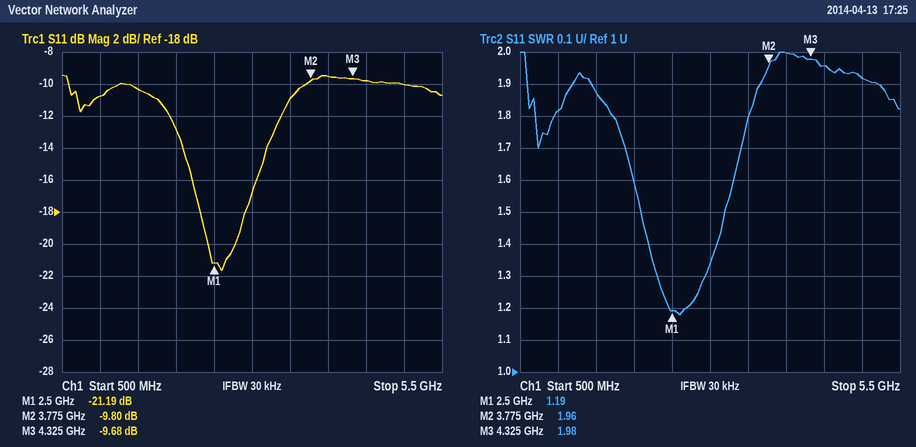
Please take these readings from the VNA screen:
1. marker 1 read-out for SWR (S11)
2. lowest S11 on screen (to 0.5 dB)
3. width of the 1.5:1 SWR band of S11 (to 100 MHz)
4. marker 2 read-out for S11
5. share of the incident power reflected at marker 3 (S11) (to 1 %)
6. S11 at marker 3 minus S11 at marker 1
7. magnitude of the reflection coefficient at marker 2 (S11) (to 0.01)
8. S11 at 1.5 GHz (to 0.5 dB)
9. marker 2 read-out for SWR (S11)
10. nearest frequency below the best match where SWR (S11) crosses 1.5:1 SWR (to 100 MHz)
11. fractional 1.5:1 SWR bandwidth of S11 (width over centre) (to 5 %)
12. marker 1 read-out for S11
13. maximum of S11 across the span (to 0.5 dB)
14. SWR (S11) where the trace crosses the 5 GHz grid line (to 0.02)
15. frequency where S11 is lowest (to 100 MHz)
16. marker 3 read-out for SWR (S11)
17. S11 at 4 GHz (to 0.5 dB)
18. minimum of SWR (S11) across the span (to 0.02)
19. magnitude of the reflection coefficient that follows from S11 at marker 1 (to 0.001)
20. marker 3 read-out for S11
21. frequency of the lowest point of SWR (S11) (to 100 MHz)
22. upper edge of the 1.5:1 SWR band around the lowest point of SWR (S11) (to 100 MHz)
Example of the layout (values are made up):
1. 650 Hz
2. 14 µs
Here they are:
1. 1.19
2. -21.5 dB
3. 1.1 GHz
4. -9.80 dB
5. 11 %
6. 11.51 dB
7. 0.32
8. -10.5 dB
9. 1.96
10. 2.1 GHz
11. 40 %
12. -21.19 dB
13. -9.5 dB
14. 1.92
15. 2.6 GHz
16. 1.98
17. -9.5 dB
18. 1.18
19. 0.087
20. -9.68 dB
21. 2.6 GHz
22. 3.2 GHz
